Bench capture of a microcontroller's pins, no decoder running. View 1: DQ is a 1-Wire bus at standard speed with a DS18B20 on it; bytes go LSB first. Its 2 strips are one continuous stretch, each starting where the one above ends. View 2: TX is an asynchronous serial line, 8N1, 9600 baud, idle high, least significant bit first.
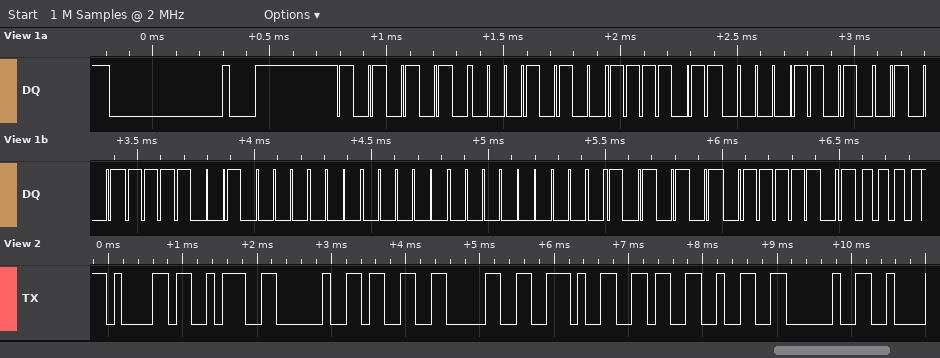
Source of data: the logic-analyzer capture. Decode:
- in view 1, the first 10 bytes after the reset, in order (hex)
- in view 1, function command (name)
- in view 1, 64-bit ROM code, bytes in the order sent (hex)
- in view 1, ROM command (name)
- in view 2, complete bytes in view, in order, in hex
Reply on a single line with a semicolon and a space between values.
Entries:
55 28 6F 58 F2 09 00 00 AA BE; Read Scratchpad; 28 6F 58 F2 09 00 00 AA; Match ROM; 61 3A 20 33 30 2E 36 32 20
